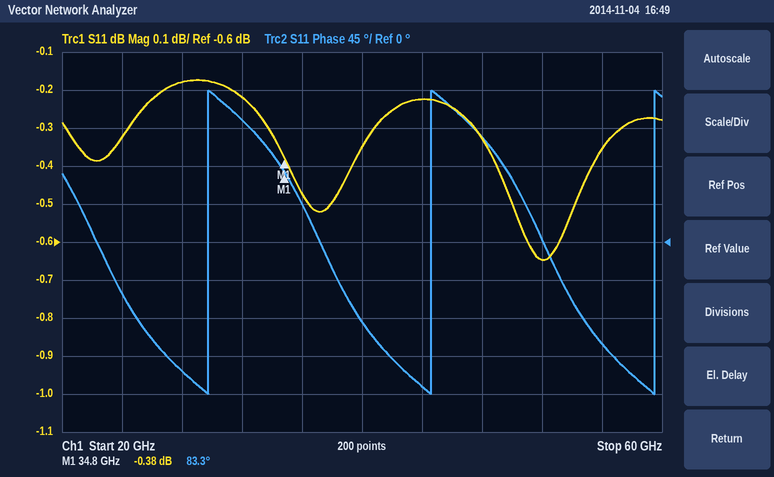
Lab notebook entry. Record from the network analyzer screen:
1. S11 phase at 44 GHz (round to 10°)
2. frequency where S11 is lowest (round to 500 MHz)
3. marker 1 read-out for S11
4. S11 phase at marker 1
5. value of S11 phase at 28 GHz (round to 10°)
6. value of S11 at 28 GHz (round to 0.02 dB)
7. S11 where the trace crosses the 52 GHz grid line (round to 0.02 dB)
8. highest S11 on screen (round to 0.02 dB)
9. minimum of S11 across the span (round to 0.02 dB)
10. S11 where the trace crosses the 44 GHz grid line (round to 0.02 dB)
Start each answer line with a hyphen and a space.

- -170°
- 52.0 GHz
- -0.38 dB
- 83.3°
- -150°
- -0.18 dB
- -0.64 dB
- -0.18 dB
- -0.64 dB
- -0.22 dB
